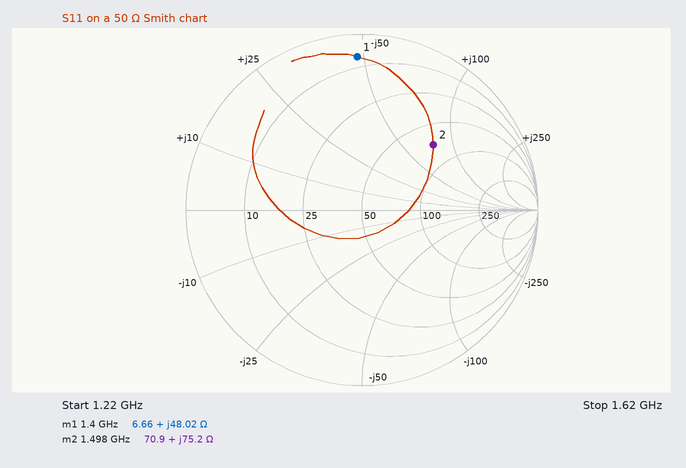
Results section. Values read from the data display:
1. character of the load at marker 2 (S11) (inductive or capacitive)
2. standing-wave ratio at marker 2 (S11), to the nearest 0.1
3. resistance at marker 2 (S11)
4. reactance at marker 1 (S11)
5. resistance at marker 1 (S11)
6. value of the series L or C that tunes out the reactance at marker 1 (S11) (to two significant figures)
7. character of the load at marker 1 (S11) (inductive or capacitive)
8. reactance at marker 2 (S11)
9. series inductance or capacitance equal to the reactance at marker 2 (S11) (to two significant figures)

inductive
3.4
70.9 Ω
+48.02 Ω
6.66 Ω
2.4 pF
inductive
+75.2 Ω
8.0 nH
